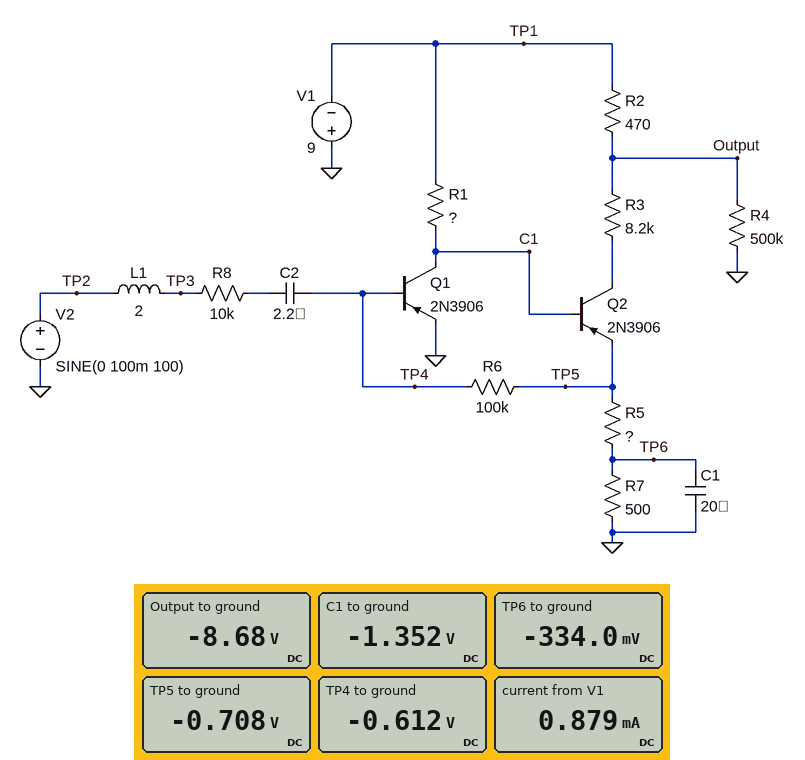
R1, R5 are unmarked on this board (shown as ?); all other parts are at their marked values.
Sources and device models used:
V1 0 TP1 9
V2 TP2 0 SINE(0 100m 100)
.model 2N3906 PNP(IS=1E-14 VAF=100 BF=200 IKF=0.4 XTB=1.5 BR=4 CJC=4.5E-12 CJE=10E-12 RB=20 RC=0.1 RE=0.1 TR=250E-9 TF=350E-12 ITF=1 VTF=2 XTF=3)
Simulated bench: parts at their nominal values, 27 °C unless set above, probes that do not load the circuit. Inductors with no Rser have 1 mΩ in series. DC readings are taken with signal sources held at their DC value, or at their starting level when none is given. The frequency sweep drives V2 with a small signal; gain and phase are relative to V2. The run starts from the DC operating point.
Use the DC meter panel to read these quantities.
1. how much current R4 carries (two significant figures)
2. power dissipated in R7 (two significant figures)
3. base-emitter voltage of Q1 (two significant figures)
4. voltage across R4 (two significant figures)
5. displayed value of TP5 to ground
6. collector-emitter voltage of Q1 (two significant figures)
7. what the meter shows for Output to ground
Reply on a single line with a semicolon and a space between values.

17 µA; 220 µW; -610 mV; 8.7 V; -0.708 V; -1.4 V; -8.68 V
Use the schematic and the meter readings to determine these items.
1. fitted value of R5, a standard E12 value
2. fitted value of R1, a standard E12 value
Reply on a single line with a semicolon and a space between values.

560 Ω; 39 kΩ
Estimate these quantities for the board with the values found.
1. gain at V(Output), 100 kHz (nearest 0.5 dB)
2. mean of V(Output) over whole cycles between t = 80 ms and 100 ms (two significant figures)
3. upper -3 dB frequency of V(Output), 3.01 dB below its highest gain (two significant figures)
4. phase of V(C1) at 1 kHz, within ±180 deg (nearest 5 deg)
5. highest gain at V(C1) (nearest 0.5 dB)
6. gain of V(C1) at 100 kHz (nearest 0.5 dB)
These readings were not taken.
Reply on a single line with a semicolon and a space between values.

-24.0 dB; -8.8 V; 840 Hz; 130 deg; 20.0 dB; -22.0 dB
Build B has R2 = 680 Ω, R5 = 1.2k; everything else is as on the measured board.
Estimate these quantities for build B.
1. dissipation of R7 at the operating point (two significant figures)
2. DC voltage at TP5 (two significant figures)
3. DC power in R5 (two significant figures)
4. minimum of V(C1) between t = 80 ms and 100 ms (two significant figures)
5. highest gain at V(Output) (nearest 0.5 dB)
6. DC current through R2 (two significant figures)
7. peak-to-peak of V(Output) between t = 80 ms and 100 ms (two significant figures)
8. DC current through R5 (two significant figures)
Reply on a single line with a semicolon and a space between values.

87 µW; -710 mV; 210 µW; -2.0 V; 14.5 dB; 430 µA; 590 mV; 420 µA
